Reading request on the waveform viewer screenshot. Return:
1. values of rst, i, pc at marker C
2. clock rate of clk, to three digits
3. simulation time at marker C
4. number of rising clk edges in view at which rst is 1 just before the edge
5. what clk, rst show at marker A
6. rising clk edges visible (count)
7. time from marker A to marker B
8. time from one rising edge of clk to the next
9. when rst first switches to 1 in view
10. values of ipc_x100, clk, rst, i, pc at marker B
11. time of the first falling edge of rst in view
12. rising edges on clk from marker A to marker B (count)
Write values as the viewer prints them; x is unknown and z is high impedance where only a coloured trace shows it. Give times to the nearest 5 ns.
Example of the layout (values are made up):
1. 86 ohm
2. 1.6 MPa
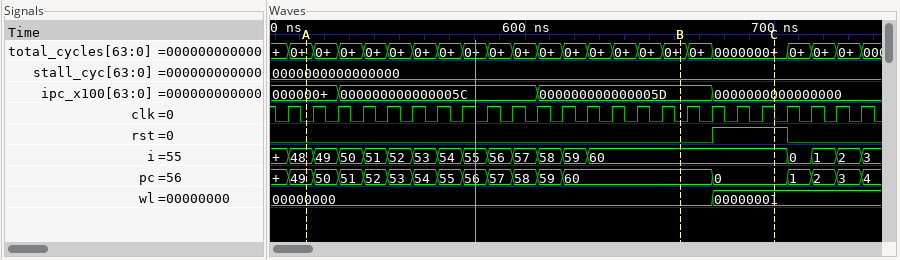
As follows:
1. rst=1, i=60, pc=0
2. 100 MHz
3. 700 ns
4. 3
5. clk=0, rst=0
6. 24
7. 150 ns
8. 10 ns
9. 675 ns
10. ipc_x100=000000000000005D, clk=0, rst=0, i=60, pc=60
11. 705 ns
12. 15
